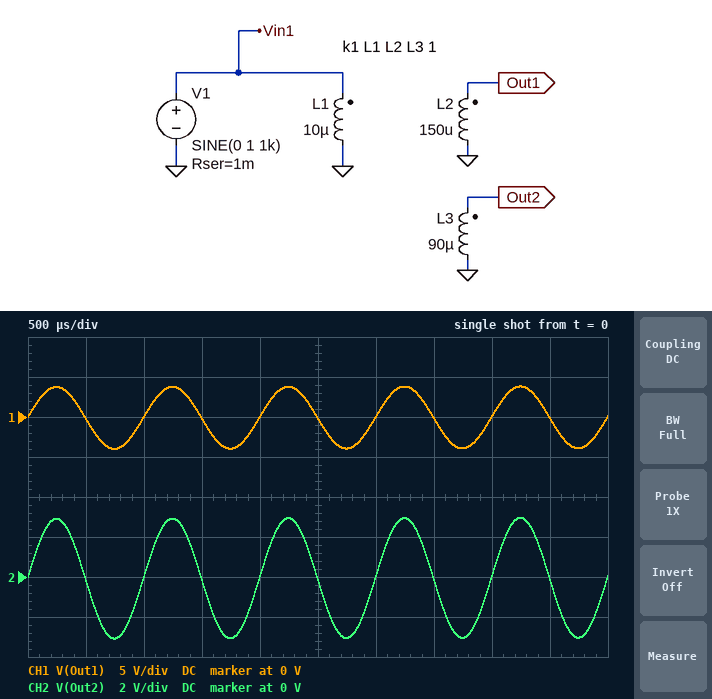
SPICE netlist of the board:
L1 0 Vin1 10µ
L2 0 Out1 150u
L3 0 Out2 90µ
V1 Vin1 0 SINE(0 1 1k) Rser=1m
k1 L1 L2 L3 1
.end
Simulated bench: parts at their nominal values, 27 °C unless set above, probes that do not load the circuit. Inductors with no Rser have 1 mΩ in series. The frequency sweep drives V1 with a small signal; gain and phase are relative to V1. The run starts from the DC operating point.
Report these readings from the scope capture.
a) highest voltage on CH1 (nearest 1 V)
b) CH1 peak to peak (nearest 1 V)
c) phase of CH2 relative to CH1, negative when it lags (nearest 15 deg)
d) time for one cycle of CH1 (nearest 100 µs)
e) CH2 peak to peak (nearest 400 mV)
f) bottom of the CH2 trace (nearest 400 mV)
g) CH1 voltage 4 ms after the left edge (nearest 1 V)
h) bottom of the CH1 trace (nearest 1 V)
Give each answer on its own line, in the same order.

4 V
8 V
0 deg
1.0 ms
6.0 V
-3.2 V
0 V
-4 V
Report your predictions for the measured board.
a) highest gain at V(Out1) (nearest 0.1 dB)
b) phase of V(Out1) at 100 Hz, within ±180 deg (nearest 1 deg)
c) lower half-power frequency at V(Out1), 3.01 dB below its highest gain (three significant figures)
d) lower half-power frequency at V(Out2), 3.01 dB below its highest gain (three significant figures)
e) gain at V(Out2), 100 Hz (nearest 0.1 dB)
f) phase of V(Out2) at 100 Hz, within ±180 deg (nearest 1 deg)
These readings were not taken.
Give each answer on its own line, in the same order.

11.8 dB
18 deg
31.8 Hz
31.8 Hz
9.1 dB
18 deg
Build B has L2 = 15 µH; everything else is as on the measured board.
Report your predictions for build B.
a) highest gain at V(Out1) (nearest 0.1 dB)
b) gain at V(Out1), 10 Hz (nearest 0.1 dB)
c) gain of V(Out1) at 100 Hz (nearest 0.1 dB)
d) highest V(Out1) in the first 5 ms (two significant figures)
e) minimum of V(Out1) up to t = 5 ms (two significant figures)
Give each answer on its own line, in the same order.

1.8 dB
-8.7 dB
1.3 dB
1.2 V
-1.3 V
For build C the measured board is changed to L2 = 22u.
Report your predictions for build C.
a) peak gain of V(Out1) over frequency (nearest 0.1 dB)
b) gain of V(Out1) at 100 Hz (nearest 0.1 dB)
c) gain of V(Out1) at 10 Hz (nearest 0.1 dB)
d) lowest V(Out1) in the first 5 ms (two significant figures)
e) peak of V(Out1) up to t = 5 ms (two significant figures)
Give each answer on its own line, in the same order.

3.4 dB
3.0 dB
-7.0 dB
-1.5 V
1.5 V
